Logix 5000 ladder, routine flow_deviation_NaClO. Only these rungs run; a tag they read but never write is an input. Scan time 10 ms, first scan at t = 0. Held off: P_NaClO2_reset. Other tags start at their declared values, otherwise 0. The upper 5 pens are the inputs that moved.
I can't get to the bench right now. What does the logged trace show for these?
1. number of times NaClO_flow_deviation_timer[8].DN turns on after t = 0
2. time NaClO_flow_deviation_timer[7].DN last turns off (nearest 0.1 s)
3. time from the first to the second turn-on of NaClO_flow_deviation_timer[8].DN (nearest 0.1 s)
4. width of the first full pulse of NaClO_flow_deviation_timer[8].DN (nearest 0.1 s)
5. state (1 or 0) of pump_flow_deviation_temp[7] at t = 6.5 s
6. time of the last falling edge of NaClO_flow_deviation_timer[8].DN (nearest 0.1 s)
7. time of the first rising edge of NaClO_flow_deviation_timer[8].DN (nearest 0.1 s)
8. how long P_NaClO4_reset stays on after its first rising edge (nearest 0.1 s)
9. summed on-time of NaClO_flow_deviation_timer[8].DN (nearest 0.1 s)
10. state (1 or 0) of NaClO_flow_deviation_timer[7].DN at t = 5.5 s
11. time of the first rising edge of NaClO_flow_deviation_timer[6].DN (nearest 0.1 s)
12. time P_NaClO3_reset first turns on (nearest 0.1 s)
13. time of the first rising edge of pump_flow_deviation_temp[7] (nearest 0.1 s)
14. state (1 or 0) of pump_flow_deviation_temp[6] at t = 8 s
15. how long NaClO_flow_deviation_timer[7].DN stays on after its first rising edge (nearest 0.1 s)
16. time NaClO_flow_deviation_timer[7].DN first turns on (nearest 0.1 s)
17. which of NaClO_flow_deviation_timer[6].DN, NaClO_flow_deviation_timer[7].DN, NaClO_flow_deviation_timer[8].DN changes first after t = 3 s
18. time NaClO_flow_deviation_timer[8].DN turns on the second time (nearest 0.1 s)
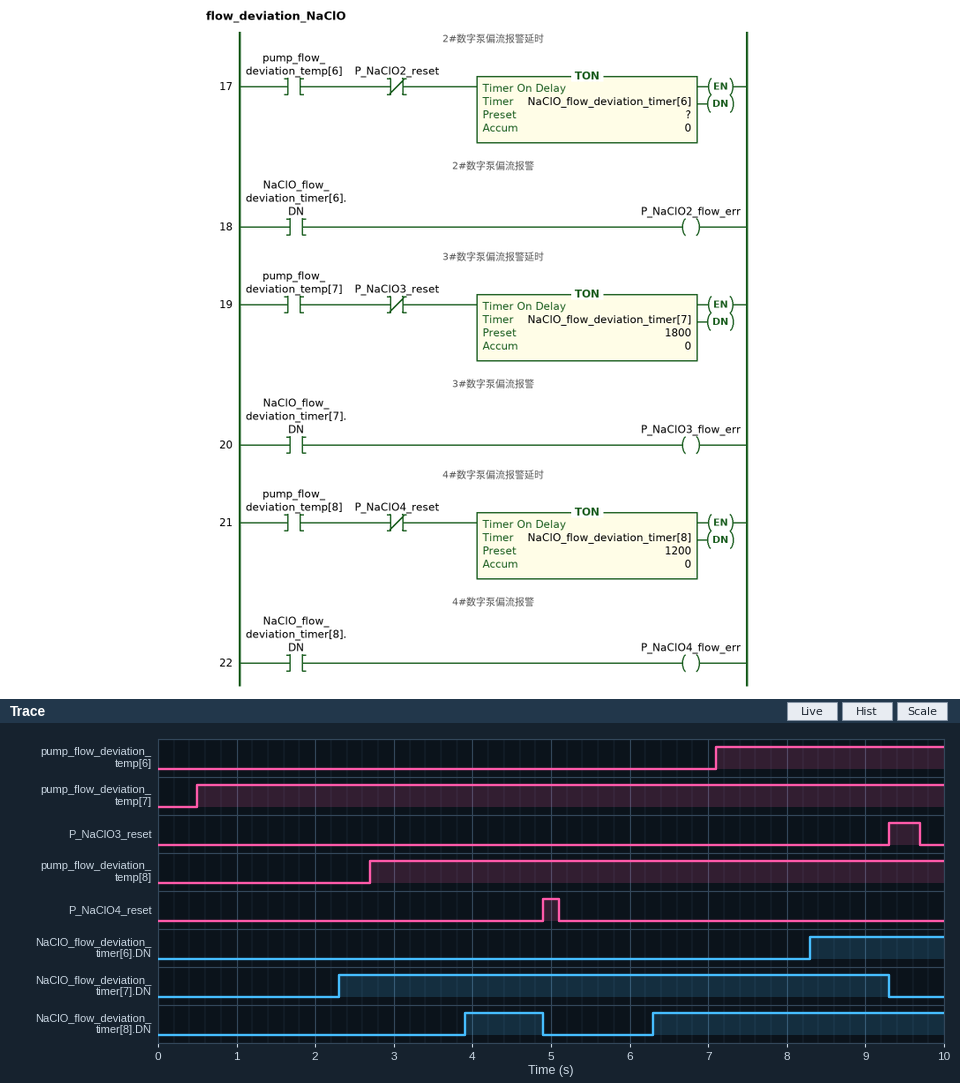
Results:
2
9.3 s
2.4 s
1.0 s
1
4.9 s
3.9 s
0.2 s
4.7 s
1
8.3 s
9.3 s
0.5 s
1
7.0 s
2.3 s
NaClO_flow_deviation_timer[8].DN
6.3 s
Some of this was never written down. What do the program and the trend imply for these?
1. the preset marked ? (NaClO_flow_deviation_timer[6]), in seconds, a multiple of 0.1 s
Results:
1.2 s
